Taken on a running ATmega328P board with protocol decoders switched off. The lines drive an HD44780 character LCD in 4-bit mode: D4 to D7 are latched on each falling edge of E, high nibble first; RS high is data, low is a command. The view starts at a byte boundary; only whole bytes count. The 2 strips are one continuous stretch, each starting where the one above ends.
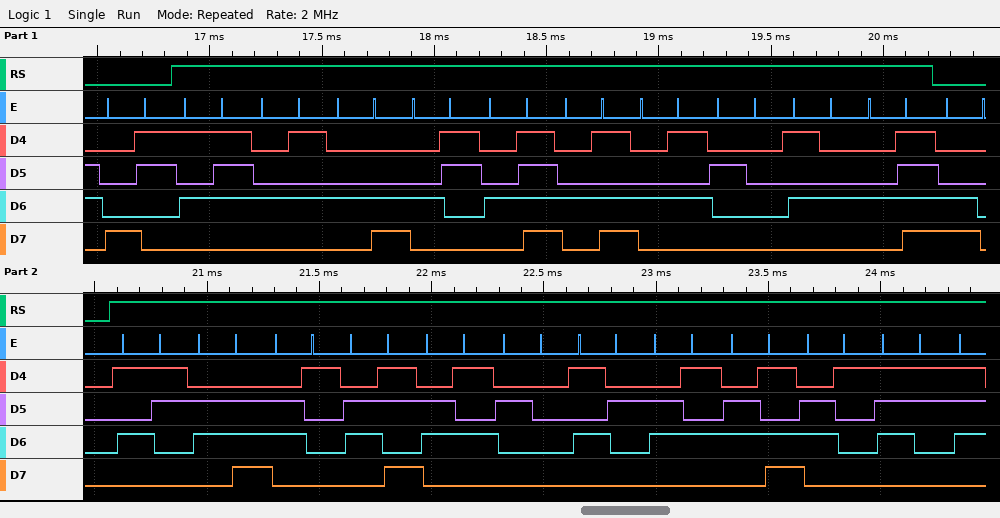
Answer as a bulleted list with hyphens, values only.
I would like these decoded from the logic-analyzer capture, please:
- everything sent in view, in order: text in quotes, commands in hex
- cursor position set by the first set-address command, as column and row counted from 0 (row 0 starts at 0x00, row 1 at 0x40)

- 0x83 "WELCOME TO" 0xC0 "Snake Remas"
- column 3, row 0
